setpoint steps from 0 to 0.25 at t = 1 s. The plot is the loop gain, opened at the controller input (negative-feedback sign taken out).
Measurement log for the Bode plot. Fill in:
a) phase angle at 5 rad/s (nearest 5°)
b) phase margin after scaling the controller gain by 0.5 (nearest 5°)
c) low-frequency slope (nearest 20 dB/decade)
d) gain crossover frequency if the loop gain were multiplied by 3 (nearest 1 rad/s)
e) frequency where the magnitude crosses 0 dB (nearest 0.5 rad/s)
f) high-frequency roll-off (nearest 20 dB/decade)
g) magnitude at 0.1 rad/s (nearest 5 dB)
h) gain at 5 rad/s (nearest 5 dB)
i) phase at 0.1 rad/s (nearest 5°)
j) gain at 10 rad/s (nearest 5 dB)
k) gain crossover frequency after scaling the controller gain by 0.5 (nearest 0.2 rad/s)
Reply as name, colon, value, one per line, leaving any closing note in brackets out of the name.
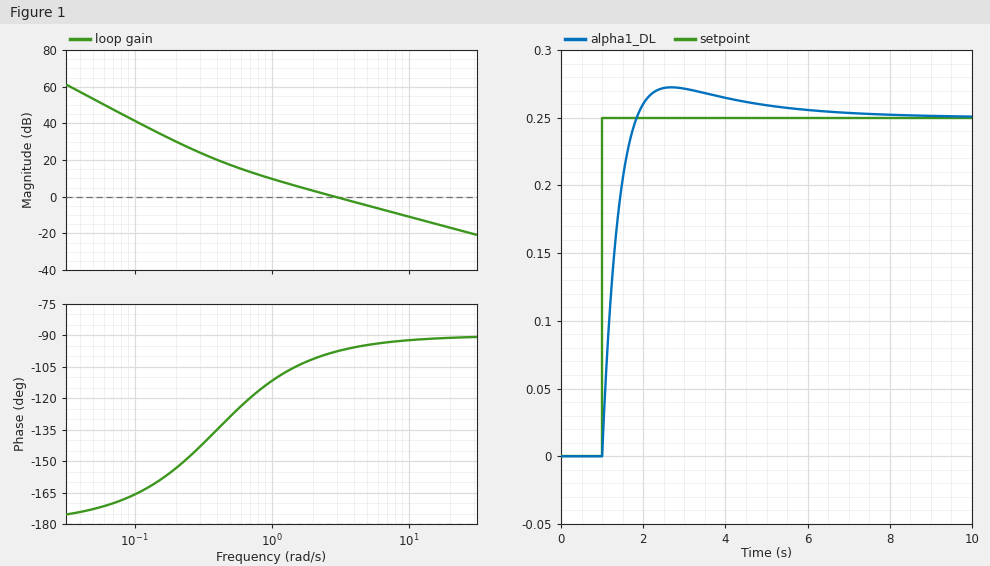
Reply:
phase angle at 5 rad/s: -95°
phase margin after scaling the controller gain by 0.5: 75°
low-frequency slope: -40 dB/decade
gain crossover frequency if the loop gain were multiplied by 3: 9 rad/s
frequency where the magnitude crosses 0 dB: 3.0 rad/s
high-frequency roll-off: -20 dB/decade
magnitude at 0.1 rad/s: 40 dB
gain at 5 rad/s: -5 dB
phase at 0.1 rad/s: -165°
gain at 10 rad/s: -10 dB
gain crossover frequency after scaling the controller gain by 0.5: 1.4 rad/s
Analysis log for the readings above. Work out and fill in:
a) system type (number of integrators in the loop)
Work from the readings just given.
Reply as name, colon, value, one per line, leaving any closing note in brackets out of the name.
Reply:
system type: 2
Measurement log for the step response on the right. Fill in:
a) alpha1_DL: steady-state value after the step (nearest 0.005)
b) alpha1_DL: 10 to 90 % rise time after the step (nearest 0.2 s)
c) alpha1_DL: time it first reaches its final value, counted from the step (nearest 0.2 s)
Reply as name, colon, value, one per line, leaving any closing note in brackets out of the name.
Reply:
alpha1_DL: steady-state value after the step: 0.250
alpha1_DL: 10 to 90 % rise time after the step: 0.6 s
alpha1_DL: time it first reaches its final value, counted from the step: 0.8 s
